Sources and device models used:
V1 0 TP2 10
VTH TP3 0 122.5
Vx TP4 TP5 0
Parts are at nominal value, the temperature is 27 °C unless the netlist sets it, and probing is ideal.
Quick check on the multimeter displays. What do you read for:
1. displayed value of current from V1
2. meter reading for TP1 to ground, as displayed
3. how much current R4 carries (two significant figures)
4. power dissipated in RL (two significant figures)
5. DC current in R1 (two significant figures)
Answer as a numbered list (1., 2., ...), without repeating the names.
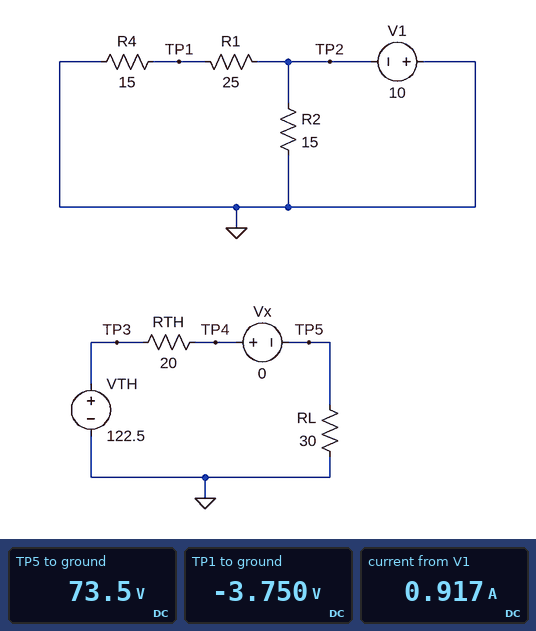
1. 0.917 A
2. -3.750 V
3. 250 mA
4. 180 W
5. 250 mA
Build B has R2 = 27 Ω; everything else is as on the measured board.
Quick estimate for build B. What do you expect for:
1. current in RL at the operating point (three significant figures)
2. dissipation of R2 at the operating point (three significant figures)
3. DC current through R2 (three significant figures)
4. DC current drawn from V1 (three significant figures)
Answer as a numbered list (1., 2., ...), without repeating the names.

1. 2.45 A
2. 3.70 W
3. 370 mA
4. 620 mA
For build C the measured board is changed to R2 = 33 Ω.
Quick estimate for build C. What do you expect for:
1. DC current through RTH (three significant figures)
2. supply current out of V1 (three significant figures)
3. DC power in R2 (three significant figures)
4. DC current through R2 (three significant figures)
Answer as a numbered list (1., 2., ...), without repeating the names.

1. 2.45 A
2. 553 mA
3. 3.03 W
4. 303 mA
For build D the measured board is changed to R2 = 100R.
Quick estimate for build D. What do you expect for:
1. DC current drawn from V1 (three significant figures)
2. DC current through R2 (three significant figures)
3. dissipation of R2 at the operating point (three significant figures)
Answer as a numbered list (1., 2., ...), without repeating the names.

1. 350 mA
2. 100 mA
3. 1.00 W
